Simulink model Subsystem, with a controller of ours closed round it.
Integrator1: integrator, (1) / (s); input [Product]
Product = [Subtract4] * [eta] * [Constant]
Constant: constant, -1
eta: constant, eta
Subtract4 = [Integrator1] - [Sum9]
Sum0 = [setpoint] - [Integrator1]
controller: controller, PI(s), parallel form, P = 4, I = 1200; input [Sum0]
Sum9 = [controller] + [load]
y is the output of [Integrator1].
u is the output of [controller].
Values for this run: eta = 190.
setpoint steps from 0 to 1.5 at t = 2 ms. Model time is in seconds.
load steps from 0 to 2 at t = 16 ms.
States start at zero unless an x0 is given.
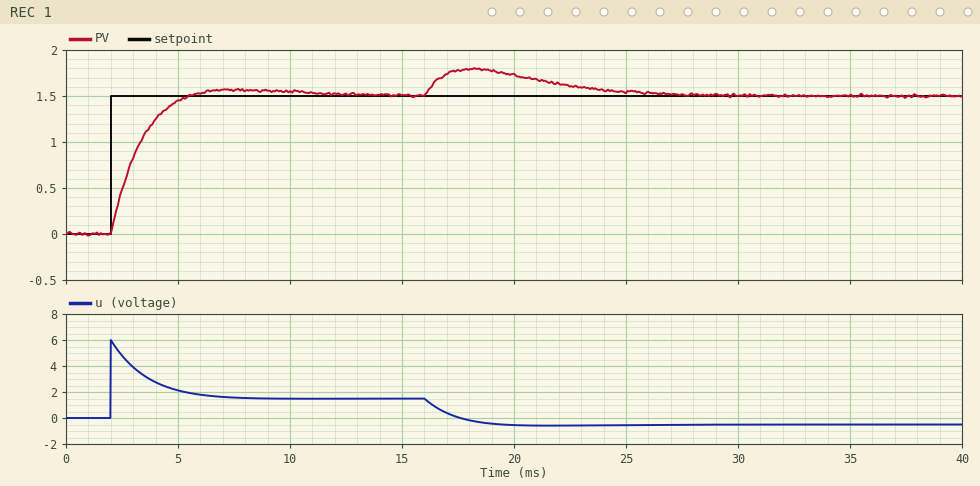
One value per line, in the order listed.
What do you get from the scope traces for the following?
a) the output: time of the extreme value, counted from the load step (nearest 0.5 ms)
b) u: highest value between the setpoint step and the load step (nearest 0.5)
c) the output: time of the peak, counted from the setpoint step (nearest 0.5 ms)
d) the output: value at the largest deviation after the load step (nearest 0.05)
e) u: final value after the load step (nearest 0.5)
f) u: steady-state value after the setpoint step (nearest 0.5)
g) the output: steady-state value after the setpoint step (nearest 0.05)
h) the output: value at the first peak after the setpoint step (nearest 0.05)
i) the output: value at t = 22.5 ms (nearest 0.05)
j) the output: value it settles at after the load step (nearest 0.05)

2.0 ms
6.0
5.5 ms
1.80
-0.5
1.5
1.50
1.55
1.60
1.50
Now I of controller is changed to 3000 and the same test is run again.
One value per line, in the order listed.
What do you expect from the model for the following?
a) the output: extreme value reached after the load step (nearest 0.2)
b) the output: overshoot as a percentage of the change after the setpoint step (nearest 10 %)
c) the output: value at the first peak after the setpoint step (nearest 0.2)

1.8
20 %
1.8
